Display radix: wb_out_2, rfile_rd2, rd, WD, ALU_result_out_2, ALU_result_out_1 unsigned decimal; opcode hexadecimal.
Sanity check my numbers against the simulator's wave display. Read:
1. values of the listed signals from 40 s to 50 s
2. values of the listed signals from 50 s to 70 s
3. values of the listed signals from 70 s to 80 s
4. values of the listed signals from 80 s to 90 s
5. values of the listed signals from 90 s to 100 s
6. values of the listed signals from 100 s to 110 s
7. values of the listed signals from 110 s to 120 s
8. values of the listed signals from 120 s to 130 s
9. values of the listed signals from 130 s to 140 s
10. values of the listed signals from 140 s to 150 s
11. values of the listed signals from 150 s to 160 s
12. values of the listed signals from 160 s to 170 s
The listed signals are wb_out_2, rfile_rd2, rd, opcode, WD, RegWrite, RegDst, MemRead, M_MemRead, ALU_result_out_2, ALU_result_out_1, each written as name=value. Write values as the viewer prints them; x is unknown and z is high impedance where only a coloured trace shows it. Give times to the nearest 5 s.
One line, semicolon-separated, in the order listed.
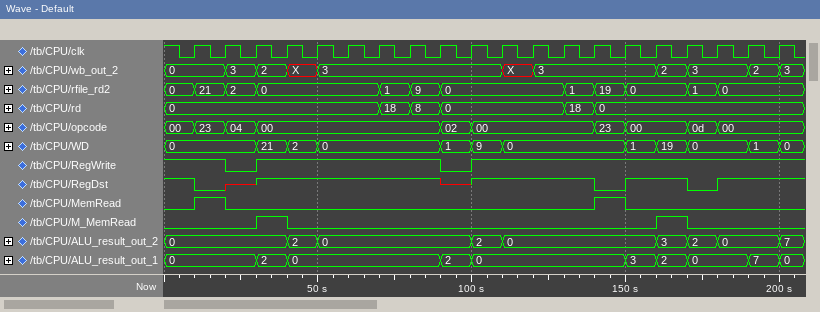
wb_out_2=X, rfile_rd2=0, rd=0, opcode=00, WD=2, RegWrite=1, RegDst=1, MemRead=0, M_MemRead=0, ALU_result_out_2=2, ALU_result_out_1=0; wb_out_2=3, rfile_rd2=0, rd=0, opcode=00, WD=0, RegWrite=1, RegDst=1, MemRead=0, M_MemRead=0, ALU_result_out_2=0, ALU_result_out_1=0; wb_out_2=3, rfile_rd2=1, rd=18, opcode=00, WD=0, RegWrite=1, RegDst=1, MemRead=0, M_MemRead=0, ALU_result_out_2=0, ALU_result_out_1=0; wb_out_2=3, rfile_rd2=9, rd=8, opcode=00, WD=0, RegWrite=1, RegDst=1, MemRead=0, M_MemRead=0, ALU_result_out_2=0, ALU_result_out_1=0; wb_out_2=3, rfile_rd2=0, rd=0, opcode=02, WD=1, RegWrite=0, RegDst=x, MemRead=0, M_MemRead=0, ALU_result_out_2=0, ALU_result_out_1=2; wb_out_2=3, rfile_rd2=0, rd=0, opcode=00, WD=9, RegWrite=1, RegDst=1, MemRead=0, M_MemRead=0, ALU_result_out_2=2, ALU_result_out_1=0; wb_out_2=X, rfile_rd2=0, rd=0, opcode=00, WD=0, RegWrite=1, RegDst=1, MemRead=0, M_MemRead=0, ALU_result_out_2=0, ALU_result_out_1=0; wb_out_2=3, rfile_rd2=0, rd=0, opcode=00, WD=0, RegWrite=1, RegDst=1, MemRead=0, M_MemRead=0, ALU_result_out_2=0, ALU_result_out_1=0; wb_out_2=3, rfile_rd2=1, rd=18, opcode=00, WD=0, RegWrite=1, RegDst=1, MemRead=0, M_MemRead=0, ALU_result_out_2=0, ALU_result_out_1=0; wb_out_2=3, rfile_rd2=19, rd=0, opcode=23, WD=0, RegWrite=1, RegDst=0, MemRead=1, M_MemRead=0, ALU_result_out_2=0, ALU_result_out_1=0; wb_out_2=3, rfile_rd2=0, rd=0, opcode=00, WD=1, RegWrite=1, RegDst=1, MemRead=0, M_MemRead=0, ALU_result_out_2=0, ALU_result_out_1=3; wb_out_2=2, rfile_rd2=0, rd=0, opcode=00, WD=19, RegWrite=1, RegDst=1, MemRead=0, M_MemRead=1, ALU_result_out_2=3, ALU_result_out_1=2
